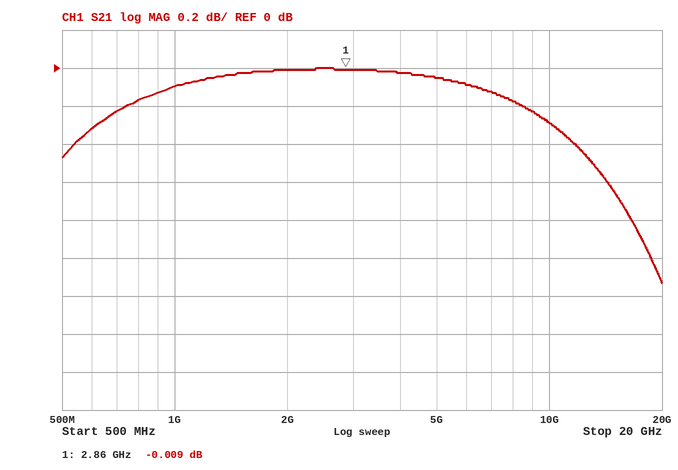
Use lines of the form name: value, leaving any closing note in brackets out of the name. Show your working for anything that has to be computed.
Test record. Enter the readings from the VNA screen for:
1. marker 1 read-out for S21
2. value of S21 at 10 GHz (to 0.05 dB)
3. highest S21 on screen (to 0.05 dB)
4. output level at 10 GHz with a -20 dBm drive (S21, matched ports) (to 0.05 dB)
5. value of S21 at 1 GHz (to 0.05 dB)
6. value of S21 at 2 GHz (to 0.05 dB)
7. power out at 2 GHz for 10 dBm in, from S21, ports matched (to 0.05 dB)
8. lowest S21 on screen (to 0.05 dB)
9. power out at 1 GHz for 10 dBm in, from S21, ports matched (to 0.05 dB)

marker 1 read-out for S21: -0.009 dB
value of S21 at 10 GHz: -0.30 dB
highest S21 on screen: 0.00 dB
output level at 10 GHz with a -20 dBm drive (S21, matched ports): -20 dBm + (-0.30 dB) = -20.30 dBm
value of S21 at 1 GHz: -0.10 dB
value of S21 at 2 GHz: 0.00 dB
power out at 2 GHz for 10 dBm in, from S21, ports matched: 10 dBm + (0.00 dB) = 10.00 dBm
lowest S21 on screen: -1.15 dB
power out at 1 GHz for 10 dBm in, from S21, ports matched: 10 dBm + (-0.10 dB) = 9.90 dBm
